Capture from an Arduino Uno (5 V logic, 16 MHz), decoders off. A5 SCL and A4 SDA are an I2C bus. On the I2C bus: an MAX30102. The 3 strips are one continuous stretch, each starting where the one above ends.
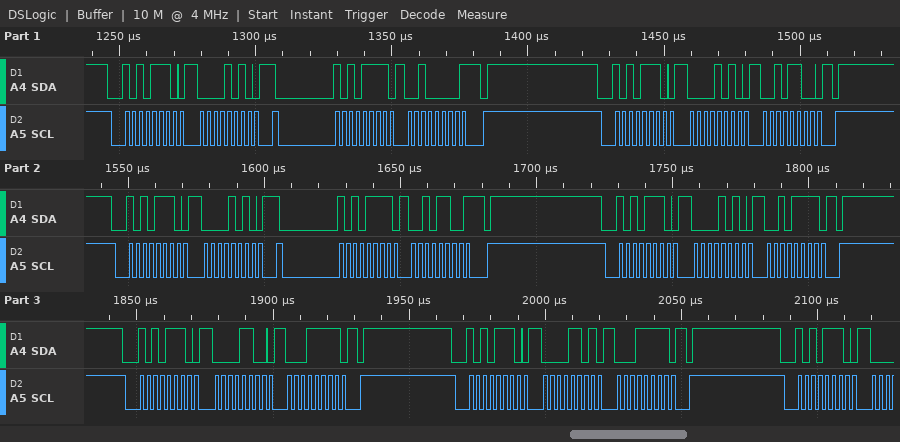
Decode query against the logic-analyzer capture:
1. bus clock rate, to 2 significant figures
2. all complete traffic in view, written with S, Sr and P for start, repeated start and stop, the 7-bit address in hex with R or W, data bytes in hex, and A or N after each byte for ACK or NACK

400 kHz
S 57W A 0A A Sr 57R A 20 N P S 57W A 0A A 2C A P S 57W A 0A A Sr 57R A 2C N P S 57W A 0A A 2F A P S 57W A 0C A 1F A P S 57W A 0D A 1F A P S 57W A
